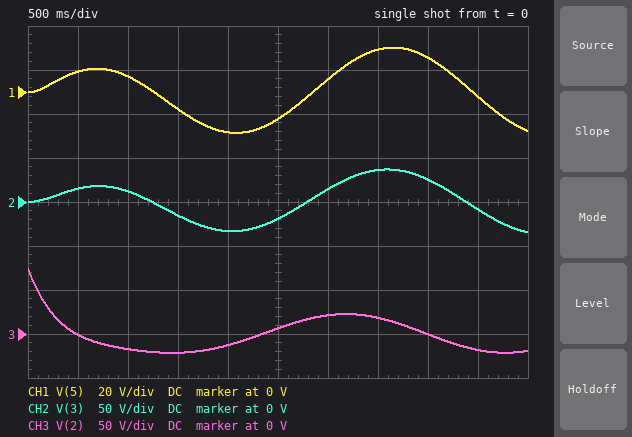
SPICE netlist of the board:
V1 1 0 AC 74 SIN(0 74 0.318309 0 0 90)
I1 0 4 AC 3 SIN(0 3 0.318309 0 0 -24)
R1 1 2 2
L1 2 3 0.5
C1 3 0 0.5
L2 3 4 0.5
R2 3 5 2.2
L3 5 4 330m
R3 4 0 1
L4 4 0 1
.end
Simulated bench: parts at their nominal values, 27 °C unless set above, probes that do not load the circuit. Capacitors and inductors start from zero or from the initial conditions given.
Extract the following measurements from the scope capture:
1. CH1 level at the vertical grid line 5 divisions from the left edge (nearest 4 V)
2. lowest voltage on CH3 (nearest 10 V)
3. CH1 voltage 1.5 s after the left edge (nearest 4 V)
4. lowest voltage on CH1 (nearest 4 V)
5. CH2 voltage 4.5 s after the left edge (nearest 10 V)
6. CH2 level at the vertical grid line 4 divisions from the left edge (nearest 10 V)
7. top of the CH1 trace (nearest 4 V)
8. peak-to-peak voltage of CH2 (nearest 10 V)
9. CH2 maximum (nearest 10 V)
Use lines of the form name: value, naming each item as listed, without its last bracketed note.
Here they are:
CH1 level at the vertical grid line 5 divisions from the left edge: -12 V
lowest voltage on CH3: -20 V
CH1 voltage 1.5 s after the left edge: -8 V
lowest voltage on CH1: -20 V
CH2 voltage 4.5 s after the left edge: -10 V
CH2 level at the vertical grid line 4 divisions from the left edge: -30 V
top of the CH1 trace: 20 V
peak-to-peak voltage of CH2: 70 V
CH2 maximum: 40 V
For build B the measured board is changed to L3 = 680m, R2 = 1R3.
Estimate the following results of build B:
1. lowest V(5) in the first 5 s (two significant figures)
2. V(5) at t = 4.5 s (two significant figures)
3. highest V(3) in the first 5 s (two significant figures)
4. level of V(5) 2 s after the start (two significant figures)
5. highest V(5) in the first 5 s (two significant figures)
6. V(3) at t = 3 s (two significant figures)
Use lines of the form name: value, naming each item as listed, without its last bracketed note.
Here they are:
lowest V(5) in the first 5 s: -25 V
V(5) at t = 4.5 s: -10 V
highest V(3) in the first 5 s: 36 V
level of V(5) 2 s after the start: -23 V
highest V(5) in the first 5 s: 25 V
V(3) at t = 3 s: 16 V
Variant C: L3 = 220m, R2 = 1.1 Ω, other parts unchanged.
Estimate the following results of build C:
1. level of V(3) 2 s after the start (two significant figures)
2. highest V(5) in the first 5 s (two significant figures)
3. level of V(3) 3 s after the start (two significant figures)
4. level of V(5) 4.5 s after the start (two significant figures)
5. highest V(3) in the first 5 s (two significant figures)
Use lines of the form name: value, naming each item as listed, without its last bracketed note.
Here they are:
level of V(3) 2 s after the start: -31 V
highest V(5) in the first 5 s: 21 V
level of V(3) 3 s after the start: 14 V
level of V(5) 4.5 s after the start: -4.9 V
highest V(3) in the first 5 s: 34 V
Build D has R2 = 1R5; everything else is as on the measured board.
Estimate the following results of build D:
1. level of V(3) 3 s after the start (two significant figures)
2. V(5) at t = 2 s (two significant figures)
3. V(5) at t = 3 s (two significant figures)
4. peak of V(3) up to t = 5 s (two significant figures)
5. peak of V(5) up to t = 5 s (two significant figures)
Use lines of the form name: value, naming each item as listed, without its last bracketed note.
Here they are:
level of V(3) 3 s after the start: 14 V
V(5) at t = 2 s: -19 V
V(5) at t = 3 s: 8.3 V
peak of V(3) up to t = 5 s: 35 V
peak of V(5) up to t = 5 s: 21 V
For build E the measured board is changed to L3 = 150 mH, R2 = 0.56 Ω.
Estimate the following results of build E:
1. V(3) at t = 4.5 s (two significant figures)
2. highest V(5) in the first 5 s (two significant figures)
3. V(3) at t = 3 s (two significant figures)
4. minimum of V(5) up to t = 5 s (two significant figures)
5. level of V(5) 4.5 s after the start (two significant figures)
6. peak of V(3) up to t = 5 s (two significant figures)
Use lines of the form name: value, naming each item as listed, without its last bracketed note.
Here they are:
V(3) at t = 4.5 s: -8.1 V
highest V(5) in the first 5 s: 22 V
V(3) at t = 3 s: 13 V
minimum of V(5) up to t = 5 s: -21 V
level of V(5) 4.5 s after the start: -7.0 V
peak of V(3) up to t = 5 s: 31 V
